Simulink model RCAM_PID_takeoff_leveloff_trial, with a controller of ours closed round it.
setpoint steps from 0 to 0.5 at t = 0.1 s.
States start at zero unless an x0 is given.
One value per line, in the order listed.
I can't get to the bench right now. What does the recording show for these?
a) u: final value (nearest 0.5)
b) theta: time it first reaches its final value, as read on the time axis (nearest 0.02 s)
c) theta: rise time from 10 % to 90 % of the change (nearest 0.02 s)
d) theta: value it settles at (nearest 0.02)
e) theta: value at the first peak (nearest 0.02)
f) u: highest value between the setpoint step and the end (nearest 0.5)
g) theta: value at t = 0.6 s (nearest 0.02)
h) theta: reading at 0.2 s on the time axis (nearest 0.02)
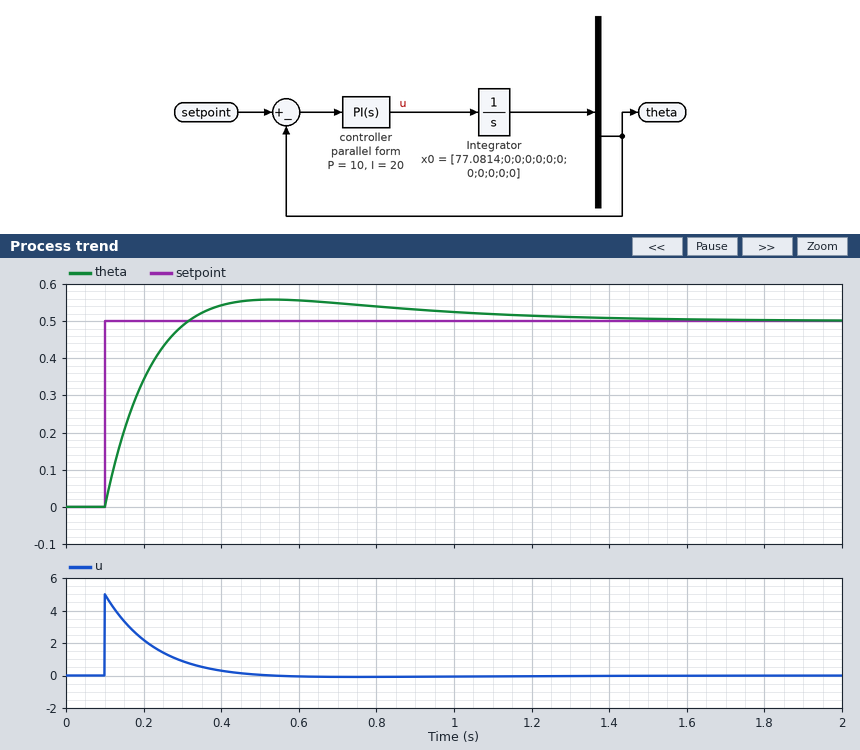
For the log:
0.0
0.32 s
0.16 s
0.50
0.56
5.0
0.56
0.34
